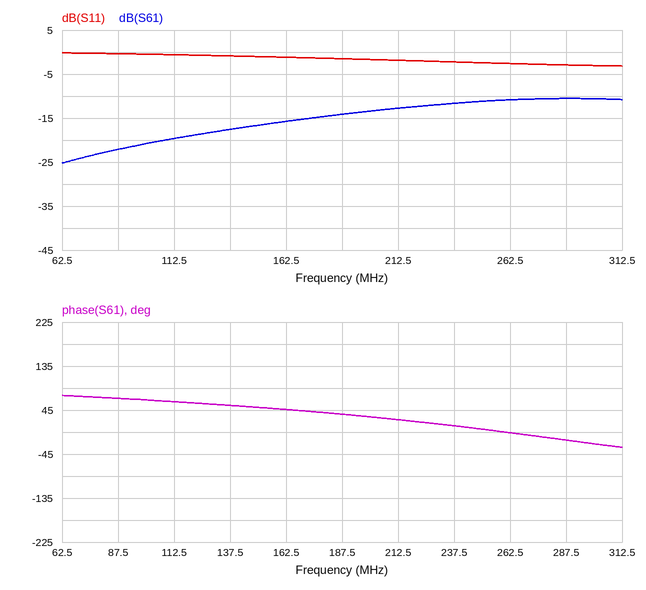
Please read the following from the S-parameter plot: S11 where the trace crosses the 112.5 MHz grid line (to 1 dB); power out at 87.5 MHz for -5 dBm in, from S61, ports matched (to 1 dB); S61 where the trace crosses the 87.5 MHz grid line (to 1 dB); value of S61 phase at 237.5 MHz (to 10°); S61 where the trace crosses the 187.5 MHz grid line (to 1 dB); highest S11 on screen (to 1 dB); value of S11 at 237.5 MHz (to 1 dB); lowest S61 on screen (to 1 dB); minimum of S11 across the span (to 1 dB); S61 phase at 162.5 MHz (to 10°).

-1 dB
-27 dBm
-22 dB
10°
-14 dB
0 dB
-2 dB
-25 dB
-3 dB
50°
